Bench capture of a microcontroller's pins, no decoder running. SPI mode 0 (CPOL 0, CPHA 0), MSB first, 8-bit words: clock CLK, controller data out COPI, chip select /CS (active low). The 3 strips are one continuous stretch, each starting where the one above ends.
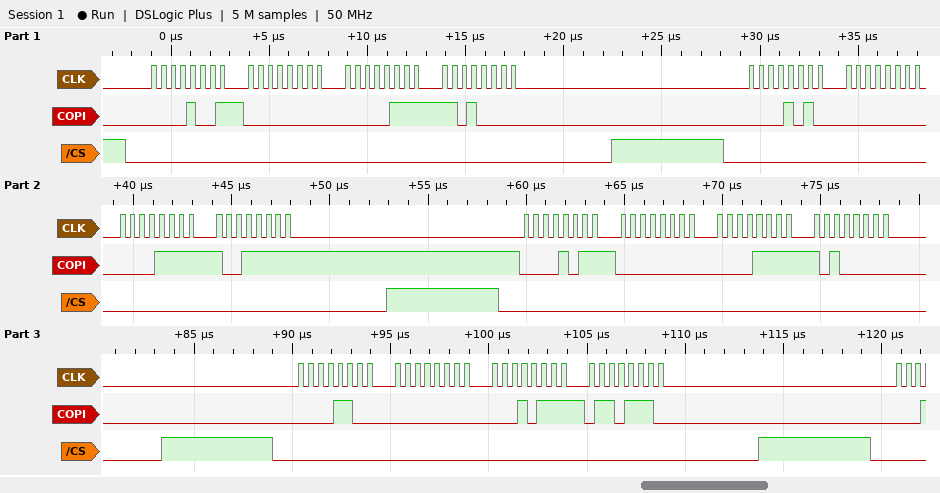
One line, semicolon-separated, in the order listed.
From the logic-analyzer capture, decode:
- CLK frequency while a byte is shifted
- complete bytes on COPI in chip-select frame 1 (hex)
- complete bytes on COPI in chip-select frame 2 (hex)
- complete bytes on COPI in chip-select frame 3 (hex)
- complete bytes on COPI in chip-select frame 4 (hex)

2 MHz; 09 00 07 D0; 0A 00 0F 9F; 0B 00 0F A0; 0C 00 17 6E
